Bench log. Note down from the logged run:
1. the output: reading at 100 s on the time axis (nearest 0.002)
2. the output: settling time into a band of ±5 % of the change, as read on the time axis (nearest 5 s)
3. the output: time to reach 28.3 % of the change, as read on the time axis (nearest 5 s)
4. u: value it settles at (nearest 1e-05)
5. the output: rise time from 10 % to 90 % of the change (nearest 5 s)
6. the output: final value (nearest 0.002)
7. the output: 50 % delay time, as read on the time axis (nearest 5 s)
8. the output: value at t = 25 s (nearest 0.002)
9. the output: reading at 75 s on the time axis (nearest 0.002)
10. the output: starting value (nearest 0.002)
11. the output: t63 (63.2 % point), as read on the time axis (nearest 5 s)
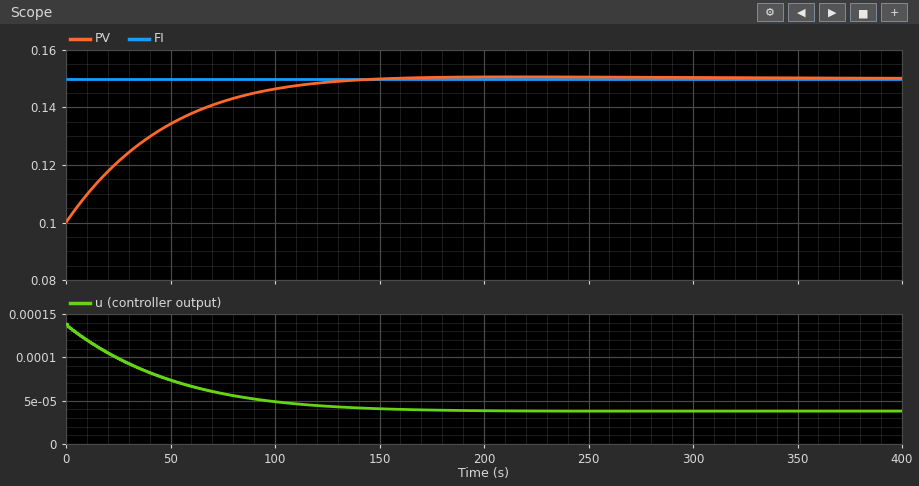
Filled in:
0.146
110 s
15 s
0.00004
85 s
0.150
30 s
0.122
0.142
0.100
45 s
